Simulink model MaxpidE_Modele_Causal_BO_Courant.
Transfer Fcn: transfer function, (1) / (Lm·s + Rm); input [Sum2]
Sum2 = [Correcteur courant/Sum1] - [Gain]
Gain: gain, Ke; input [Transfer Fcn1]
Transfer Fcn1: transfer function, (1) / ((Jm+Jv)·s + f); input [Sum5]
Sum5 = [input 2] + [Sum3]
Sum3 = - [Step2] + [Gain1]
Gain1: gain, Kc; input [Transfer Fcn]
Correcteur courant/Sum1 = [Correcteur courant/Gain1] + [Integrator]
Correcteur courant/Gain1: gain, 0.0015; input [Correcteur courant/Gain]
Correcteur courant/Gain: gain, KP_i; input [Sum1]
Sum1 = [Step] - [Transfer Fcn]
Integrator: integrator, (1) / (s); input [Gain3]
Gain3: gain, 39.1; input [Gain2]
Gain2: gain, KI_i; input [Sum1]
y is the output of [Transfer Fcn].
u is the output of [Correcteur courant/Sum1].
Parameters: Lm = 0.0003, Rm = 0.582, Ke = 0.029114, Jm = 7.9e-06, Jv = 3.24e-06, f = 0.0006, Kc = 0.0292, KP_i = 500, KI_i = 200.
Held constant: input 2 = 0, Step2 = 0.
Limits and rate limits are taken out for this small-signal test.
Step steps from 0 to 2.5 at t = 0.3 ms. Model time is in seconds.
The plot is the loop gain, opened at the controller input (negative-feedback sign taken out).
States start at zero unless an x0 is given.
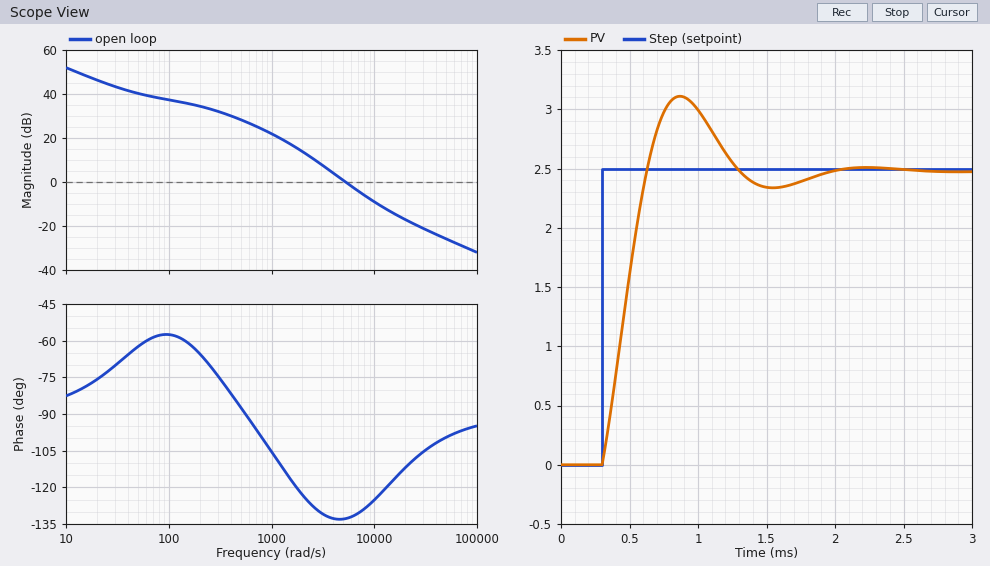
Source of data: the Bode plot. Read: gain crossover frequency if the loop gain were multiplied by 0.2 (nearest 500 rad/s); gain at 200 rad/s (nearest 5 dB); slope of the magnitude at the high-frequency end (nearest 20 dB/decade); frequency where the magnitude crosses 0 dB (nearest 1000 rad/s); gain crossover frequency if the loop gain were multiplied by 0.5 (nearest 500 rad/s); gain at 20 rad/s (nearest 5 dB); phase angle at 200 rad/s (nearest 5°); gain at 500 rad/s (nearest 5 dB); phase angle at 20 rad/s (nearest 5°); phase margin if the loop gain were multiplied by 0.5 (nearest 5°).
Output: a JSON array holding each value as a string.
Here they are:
["2000 rad/s", "35 dB", "-20 dB/decade", "5000 rad/s", "3500 rad/s", "45 dB", "-65°", "30 dB", "-75°", "50°"]
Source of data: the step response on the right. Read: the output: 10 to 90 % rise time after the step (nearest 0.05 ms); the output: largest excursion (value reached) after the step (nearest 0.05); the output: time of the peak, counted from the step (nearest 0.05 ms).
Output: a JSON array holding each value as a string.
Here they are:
["0.25 ms", "3.10", "0.55 ms"]
